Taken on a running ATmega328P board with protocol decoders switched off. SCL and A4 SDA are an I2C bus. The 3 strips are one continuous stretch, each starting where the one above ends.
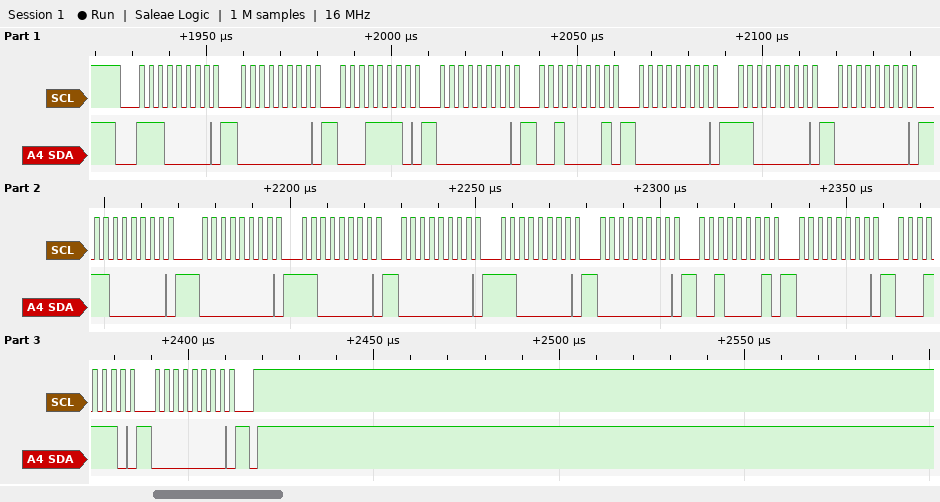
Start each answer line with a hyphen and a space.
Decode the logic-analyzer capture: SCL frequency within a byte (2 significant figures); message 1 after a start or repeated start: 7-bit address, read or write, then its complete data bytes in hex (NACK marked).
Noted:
- 400 kHz
- 0x70 write: 00 1E 00 21 00 C0 00 C0 00 C0 00 C0 00 21 00 1E 00
